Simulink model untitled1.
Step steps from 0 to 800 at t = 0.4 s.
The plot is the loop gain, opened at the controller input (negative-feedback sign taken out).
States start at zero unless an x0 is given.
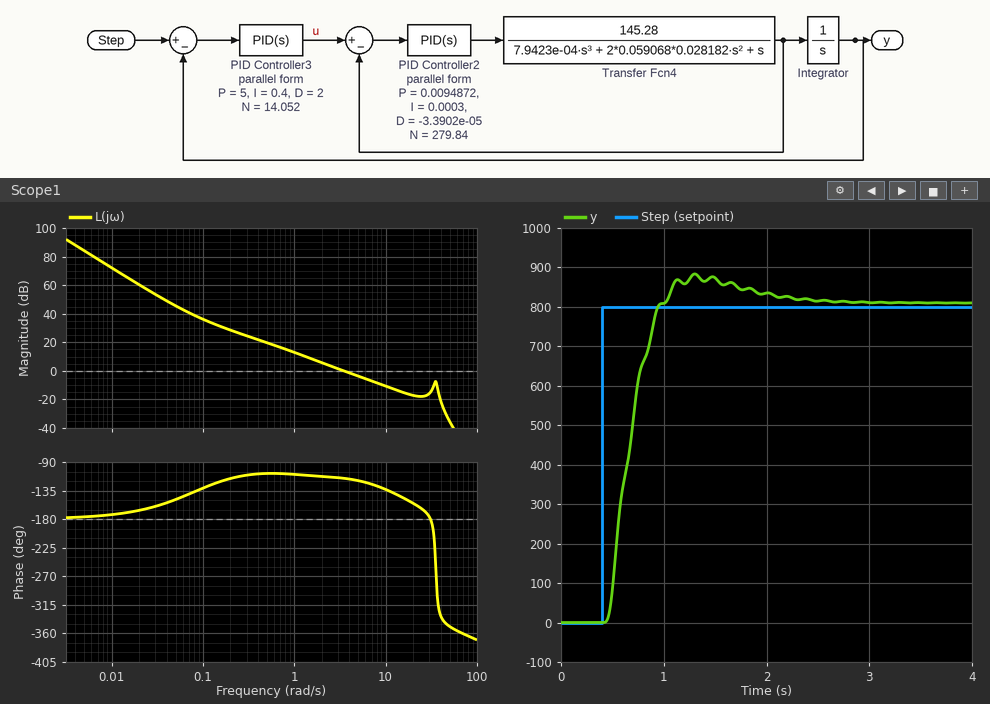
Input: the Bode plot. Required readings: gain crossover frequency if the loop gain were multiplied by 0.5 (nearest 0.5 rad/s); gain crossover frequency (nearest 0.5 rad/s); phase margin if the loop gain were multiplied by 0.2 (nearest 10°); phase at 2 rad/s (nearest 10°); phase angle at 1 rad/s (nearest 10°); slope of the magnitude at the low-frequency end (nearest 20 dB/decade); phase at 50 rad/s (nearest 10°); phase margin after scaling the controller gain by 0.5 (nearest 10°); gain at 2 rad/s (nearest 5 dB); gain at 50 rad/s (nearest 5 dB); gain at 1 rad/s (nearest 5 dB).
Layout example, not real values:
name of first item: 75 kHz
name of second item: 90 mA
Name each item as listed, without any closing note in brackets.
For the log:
gain crossover frequency if the loop gain were multiplied by 0.5: 2.0 rad/s
gain crossover frequency: 3.5 rad/s
phase margin if the loop gain were multiplied by 0.2: 70°
phase at 2 rad/s: -110°
phase angle at 1 rad/s: -110°
slope of the magnitude at the low-frequency end: -40 dB/decade
phase at 50 rad/s: -350°
phase margin after scaling the controller gain by 0.5: 70°
gain at 2 rad/s: 5 dB
gain at 50 rad/s: -35 dB
gain at 1 rad/s: 15 dB
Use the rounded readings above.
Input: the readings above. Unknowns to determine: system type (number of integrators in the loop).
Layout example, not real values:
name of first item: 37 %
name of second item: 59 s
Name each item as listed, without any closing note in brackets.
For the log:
system type: 2
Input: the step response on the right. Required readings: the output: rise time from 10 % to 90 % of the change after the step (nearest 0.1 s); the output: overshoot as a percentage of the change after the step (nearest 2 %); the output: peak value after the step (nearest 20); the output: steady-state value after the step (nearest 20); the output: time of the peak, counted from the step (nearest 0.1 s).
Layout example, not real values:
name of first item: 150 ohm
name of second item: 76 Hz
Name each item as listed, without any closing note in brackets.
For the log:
the output: rise time from 10 % to 90 % of the change after the step: 0.4 s
the output: overshoot as a percentage of the change after the step: 10 %
the output: peak value after the step: 880
the output: steady-state value after the step: 800
the output: time of the peak, counted from the step: 0.9 s
